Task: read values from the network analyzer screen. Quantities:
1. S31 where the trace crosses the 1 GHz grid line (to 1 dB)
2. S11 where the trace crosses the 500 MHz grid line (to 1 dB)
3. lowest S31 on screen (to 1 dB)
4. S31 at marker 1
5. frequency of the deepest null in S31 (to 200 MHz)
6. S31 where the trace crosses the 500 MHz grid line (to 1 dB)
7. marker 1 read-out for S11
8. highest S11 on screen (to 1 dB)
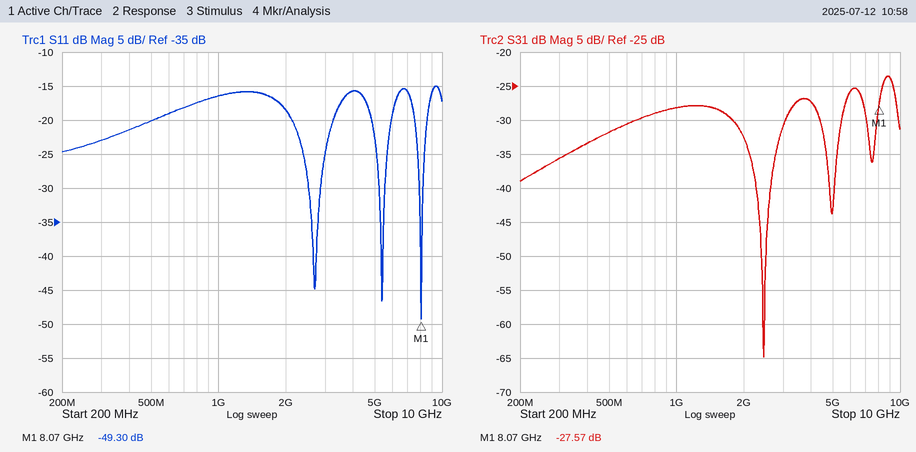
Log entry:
-28 dB
-20 dB
-65 dB
-27.57 dB
2.4 GHz
-32 dB
-49.30 dB
-15 dB
